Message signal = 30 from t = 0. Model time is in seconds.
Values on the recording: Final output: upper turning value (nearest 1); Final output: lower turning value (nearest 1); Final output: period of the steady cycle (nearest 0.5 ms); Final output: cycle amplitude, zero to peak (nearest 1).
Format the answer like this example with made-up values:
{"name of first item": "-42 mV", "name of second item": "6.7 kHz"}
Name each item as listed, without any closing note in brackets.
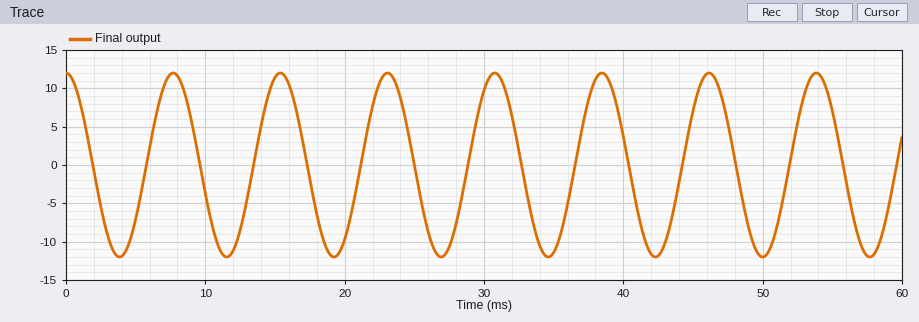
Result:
{"Final output: upper turning value": "12", "Final output: lower turning value": "-12", "Final output: period of the steady cycle": "7.5 ms", "Final output: cycle amplitude, zero to peak": "12"}
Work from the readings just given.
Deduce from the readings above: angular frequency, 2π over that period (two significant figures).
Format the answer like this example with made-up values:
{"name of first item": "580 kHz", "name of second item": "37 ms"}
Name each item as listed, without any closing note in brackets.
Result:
{"angular frequency, 2π over that period": "0.84 rad/ms"}
